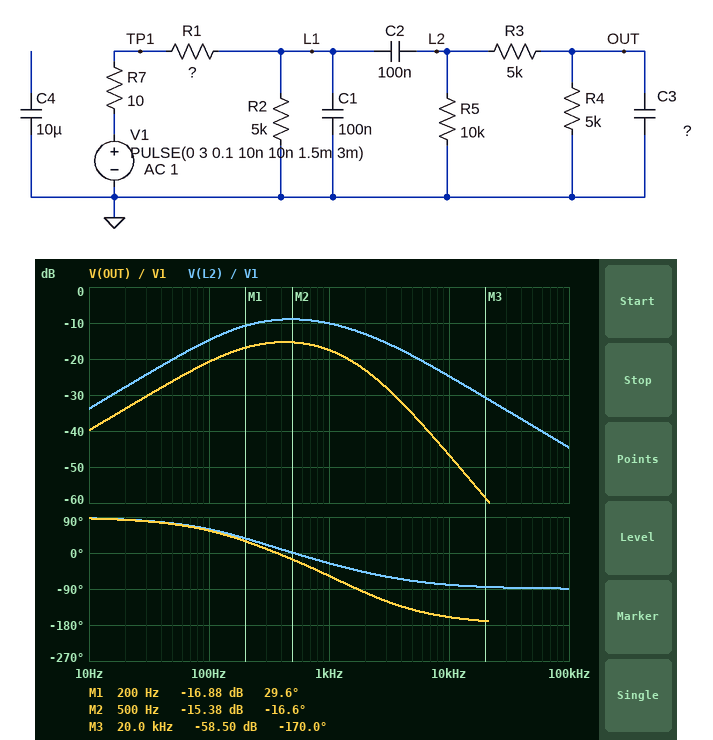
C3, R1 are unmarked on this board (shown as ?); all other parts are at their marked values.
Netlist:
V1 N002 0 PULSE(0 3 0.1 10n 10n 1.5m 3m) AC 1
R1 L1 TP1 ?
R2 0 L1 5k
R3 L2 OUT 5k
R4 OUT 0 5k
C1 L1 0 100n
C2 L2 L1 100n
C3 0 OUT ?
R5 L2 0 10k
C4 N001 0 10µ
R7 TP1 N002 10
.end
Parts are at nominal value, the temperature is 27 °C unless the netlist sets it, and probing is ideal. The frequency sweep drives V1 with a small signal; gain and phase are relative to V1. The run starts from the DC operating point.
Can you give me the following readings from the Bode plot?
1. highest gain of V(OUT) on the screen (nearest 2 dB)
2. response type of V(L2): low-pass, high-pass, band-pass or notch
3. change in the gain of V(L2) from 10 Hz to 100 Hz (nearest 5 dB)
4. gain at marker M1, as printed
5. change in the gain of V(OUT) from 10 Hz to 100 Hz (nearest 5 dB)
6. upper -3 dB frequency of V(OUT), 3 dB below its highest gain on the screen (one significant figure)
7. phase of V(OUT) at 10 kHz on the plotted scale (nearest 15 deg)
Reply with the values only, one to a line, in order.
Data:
-16 dB
band-pass
20 dB
-16.88 dB
20 dB
1 kHz
-165 deg
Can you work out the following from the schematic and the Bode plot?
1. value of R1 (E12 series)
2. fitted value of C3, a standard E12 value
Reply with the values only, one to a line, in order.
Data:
2.7 kΩ
39 nF
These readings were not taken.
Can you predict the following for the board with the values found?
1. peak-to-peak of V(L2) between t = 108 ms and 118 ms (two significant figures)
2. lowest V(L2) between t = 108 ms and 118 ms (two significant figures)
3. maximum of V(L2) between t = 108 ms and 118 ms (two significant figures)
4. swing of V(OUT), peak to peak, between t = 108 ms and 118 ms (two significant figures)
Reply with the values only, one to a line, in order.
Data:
1.5 V
-730 mV
730 mV
690 mV
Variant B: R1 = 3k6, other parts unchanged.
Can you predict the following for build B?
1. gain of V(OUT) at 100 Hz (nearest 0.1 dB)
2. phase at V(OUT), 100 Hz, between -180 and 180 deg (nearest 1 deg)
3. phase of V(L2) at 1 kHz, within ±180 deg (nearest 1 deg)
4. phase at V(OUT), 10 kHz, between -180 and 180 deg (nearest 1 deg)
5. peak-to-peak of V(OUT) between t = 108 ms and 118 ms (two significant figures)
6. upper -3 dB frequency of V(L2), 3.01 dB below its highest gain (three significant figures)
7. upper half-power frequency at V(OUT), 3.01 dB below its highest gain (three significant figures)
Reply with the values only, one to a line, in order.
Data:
-21.9 dB
54 deg
-29 deg
-161 deg
560 mV
1.44 kHz
1.07 kHz
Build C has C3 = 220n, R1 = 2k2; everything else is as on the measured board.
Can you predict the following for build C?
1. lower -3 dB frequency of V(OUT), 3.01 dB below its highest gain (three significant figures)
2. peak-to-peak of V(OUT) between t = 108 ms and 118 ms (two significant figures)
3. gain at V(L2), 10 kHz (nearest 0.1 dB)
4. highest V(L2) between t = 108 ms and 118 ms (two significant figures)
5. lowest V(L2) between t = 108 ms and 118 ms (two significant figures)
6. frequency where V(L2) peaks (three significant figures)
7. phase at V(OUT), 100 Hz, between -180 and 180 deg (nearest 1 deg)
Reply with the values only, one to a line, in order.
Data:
87.5 Hz
360 mV
-23.0 dB
760 mV
-760 mV
683 Hz
37 deg
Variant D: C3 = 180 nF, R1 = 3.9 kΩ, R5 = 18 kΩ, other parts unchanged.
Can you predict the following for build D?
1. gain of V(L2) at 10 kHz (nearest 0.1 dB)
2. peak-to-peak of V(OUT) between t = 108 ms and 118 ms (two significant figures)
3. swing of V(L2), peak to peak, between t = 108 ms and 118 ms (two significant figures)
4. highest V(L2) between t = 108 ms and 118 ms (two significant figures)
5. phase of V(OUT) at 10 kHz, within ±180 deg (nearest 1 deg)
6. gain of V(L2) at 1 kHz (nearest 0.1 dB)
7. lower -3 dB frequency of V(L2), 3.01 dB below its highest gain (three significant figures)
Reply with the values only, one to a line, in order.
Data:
-27.9 dB
320 mV
1.0 V
510 mV
-169 deg
-12.6 dB
109 Hz
